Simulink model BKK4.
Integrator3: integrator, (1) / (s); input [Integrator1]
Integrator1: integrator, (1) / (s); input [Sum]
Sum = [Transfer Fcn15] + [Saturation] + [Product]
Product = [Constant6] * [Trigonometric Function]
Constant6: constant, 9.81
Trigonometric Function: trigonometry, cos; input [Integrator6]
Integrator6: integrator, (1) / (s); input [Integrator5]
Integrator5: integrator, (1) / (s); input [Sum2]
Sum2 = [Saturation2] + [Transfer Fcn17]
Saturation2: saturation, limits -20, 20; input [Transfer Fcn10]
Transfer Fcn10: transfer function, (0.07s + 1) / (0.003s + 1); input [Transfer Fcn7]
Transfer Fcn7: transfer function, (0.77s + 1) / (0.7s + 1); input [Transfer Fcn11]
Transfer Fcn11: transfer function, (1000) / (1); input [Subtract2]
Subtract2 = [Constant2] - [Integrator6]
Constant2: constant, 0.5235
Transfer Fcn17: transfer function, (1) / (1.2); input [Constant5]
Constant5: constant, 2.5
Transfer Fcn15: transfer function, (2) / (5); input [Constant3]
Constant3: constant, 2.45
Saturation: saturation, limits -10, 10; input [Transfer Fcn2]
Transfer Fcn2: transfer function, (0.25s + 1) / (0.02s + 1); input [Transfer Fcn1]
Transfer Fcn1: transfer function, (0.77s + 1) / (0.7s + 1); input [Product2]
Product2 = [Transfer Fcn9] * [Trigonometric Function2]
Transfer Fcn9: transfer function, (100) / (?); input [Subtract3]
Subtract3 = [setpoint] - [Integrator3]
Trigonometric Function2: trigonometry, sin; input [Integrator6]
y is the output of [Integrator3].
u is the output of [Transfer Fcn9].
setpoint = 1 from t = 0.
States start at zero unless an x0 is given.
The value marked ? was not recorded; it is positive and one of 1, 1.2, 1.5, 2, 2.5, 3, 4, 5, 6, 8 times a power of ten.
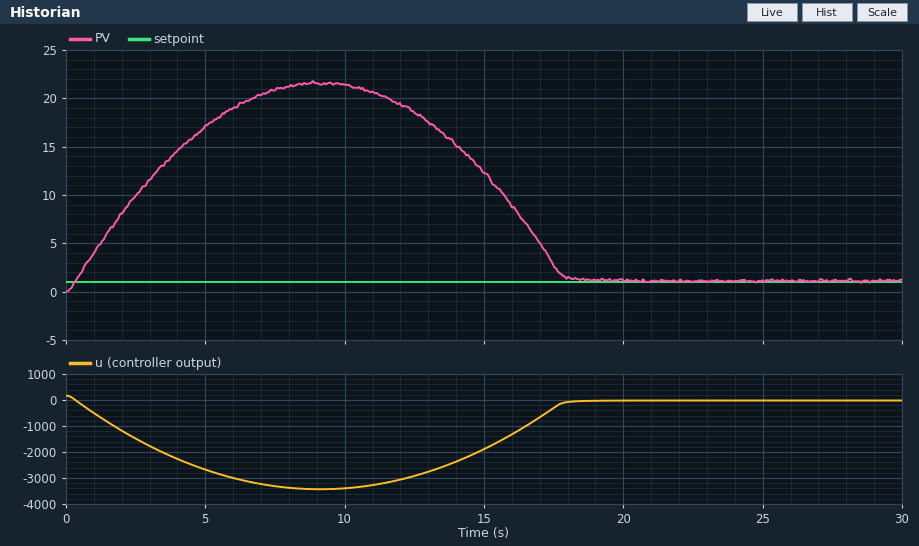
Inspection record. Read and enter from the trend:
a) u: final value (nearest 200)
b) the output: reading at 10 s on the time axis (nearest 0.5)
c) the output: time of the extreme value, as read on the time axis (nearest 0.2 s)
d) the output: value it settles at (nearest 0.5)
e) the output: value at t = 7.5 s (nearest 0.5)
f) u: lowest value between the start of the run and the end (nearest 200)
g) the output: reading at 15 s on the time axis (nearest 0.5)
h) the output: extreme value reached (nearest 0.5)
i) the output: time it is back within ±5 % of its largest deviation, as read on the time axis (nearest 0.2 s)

0
21.5
9.2 s
1.0
21.0
-3400
12.5
21.5
17.6 s
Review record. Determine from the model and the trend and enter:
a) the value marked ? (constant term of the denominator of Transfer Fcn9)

0.6
